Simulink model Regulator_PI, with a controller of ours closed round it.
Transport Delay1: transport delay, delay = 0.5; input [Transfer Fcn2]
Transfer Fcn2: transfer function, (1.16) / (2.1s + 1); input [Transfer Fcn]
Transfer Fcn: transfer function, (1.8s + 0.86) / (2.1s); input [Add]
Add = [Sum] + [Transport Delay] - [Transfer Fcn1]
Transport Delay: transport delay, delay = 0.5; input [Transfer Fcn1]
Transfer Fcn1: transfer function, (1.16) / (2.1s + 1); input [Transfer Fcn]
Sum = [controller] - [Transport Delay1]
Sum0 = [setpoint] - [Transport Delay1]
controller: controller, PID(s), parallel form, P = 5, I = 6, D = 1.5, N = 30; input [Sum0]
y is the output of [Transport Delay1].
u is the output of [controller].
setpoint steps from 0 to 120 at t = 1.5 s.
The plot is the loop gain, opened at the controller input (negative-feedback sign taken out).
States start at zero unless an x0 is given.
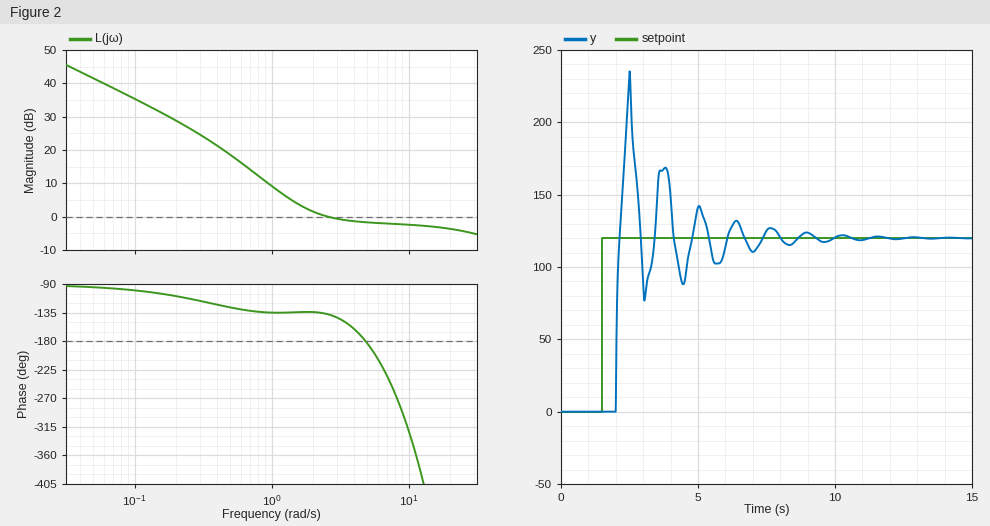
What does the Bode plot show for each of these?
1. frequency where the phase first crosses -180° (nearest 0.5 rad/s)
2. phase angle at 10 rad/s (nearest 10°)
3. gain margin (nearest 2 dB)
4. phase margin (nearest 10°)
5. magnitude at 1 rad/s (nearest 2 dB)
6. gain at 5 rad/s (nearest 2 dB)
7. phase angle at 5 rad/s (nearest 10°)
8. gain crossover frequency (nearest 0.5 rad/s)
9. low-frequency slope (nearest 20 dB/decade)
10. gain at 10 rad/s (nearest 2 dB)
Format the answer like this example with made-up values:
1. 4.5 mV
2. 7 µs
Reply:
1. 5.0 rad/s
2. -320°
3. 2 dB
4. 40°
5. 10 dB
6. -2 dB
7. -180°
8. 2.5 rad/s
9. -20 dB/decade
10. -2 dB
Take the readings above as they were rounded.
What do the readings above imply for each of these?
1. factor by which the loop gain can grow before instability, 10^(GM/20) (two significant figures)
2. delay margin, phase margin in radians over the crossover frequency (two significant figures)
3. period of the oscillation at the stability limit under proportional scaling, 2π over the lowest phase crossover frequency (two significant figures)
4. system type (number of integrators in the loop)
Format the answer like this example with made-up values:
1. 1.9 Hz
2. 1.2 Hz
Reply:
1. 1.3
2. 0.28 s
3. 1.3 s
4. 1
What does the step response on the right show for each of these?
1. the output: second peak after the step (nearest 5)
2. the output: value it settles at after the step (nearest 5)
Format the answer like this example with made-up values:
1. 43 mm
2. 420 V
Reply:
1. 170
2. 120
